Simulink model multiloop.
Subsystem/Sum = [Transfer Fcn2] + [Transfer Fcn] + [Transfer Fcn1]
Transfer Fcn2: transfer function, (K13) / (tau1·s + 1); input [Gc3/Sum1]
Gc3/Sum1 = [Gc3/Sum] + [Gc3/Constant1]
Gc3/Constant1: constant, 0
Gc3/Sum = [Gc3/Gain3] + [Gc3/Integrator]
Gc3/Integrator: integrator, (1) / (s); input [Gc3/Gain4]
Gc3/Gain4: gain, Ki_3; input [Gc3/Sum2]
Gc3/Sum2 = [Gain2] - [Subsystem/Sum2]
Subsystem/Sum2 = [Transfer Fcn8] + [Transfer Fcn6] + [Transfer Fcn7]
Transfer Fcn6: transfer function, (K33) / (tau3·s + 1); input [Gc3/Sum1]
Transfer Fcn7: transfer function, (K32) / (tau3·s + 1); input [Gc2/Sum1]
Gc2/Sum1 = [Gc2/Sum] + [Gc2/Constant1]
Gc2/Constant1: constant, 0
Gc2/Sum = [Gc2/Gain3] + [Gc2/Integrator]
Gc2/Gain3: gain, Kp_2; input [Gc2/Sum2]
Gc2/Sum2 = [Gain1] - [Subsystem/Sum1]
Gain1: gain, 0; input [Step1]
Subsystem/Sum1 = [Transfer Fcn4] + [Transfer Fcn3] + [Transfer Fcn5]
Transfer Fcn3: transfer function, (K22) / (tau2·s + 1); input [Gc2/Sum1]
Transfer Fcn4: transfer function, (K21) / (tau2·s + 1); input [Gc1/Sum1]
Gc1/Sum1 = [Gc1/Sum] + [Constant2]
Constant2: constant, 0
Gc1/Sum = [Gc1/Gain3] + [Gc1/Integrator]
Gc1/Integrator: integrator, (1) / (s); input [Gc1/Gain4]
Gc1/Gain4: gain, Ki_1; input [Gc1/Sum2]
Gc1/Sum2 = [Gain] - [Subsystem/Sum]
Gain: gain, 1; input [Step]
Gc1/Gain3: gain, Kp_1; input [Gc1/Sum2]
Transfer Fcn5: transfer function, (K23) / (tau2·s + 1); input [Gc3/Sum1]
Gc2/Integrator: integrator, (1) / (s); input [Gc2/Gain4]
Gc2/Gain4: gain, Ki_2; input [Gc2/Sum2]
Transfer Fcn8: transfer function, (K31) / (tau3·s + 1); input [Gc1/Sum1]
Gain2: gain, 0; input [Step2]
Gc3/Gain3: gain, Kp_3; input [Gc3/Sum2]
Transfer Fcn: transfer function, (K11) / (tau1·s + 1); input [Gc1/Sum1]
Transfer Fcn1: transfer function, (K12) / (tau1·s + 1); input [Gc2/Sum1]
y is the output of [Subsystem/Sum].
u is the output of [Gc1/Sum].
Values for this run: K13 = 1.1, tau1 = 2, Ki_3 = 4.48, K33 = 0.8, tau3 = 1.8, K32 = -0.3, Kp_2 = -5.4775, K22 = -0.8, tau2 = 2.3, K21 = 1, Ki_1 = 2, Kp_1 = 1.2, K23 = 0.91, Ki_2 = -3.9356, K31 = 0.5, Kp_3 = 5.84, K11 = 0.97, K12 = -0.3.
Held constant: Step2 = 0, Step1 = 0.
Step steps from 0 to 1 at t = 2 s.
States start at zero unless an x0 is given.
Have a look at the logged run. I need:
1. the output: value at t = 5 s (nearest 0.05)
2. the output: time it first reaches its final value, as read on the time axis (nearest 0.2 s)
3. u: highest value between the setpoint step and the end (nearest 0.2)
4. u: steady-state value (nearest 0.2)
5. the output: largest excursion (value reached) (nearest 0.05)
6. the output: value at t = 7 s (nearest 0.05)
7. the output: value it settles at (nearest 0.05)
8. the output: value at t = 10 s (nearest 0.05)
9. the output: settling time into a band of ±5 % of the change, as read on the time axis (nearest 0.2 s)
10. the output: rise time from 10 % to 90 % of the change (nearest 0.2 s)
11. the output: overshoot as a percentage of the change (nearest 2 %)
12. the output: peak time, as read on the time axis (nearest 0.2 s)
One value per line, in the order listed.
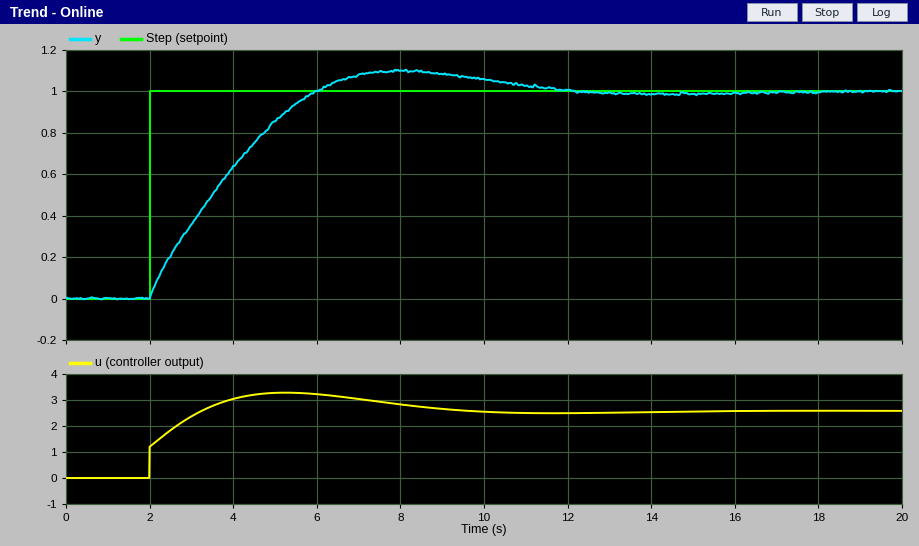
0.85
6.0 s
3.2
2.6
1.10
1.10
1.00
1.05
10.2 s
3.0 s
10 %
8.0 s
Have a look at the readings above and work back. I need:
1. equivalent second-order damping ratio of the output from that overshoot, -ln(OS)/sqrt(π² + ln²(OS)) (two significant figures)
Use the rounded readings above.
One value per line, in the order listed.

0.59
